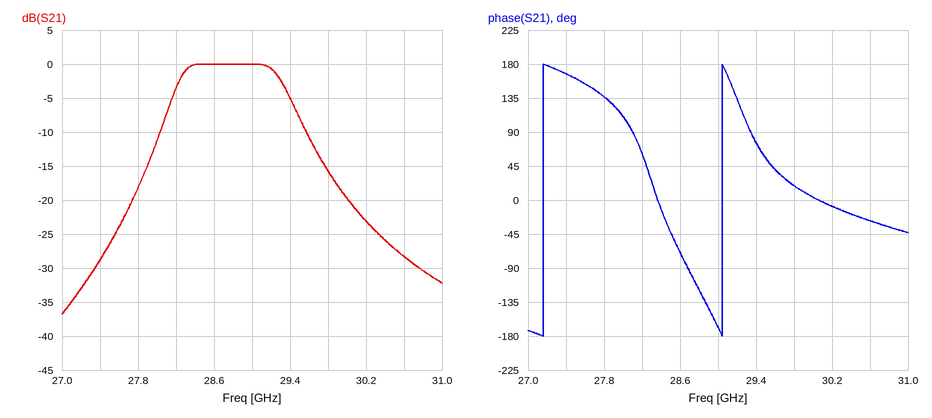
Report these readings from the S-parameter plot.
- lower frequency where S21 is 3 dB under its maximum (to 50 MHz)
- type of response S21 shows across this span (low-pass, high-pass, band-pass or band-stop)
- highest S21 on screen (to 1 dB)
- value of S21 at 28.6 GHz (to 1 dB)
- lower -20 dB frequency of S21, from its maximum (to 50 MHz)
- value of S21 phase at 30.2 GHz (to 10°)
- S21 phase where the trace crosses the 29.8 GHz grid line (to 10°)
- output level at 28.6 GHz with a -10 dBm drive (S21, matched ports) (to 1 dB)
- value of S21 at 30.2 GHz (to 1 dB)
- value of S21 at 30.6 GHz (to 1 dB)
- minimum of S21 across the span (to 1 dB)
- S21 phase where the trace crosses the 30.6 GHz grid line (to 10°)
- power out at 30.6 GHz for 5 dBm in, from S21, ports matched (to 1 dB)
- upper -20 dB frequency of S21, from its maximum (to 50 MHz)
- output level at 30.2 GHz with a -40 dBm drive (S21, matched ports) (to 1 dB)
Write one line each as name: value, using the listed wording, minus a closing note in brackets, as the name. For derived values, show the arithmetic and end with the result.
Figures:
lower frequency where S21 is 3 dB under its maximum: 28.20 GHz
type of response S21 shows across this span: band-pass
highest S21 on screen: 0 dB
value of S21 at 28.6 GHz: 0 dB
lower -20 dB frequency of S21, from its maximum: 27.75 GHz
value of S21 phase at 30.2 GHz: -10°
S21 phase where the trace crosses the 29.8 GHz grid line: 20°
output level at 28.6 GHz with a -10 dBm drive (S21, matched ports): -10 dBm + (0 dB) = -10 dBm
value of S21 at 30.2 GHz: -23 dB
value of S21 at 30.6 GHz: -28 dB
minimum of S21 across the span: -37 dB
S21 phase where the trace crosses the 30.6 GHz grid line: -30°
power out at 30.6 GHz for 5 dBm in, from S21, ports matched: 5 dBm + (-28 dB) = -23 dBm
upper -20 dB frequency of S21, from its maximum: 30.00 GHz
output level at 30.2 GHz with a -40 dBm drive (S21, matched ports): -40 dBm + (-23 dB) = -63 dBm
